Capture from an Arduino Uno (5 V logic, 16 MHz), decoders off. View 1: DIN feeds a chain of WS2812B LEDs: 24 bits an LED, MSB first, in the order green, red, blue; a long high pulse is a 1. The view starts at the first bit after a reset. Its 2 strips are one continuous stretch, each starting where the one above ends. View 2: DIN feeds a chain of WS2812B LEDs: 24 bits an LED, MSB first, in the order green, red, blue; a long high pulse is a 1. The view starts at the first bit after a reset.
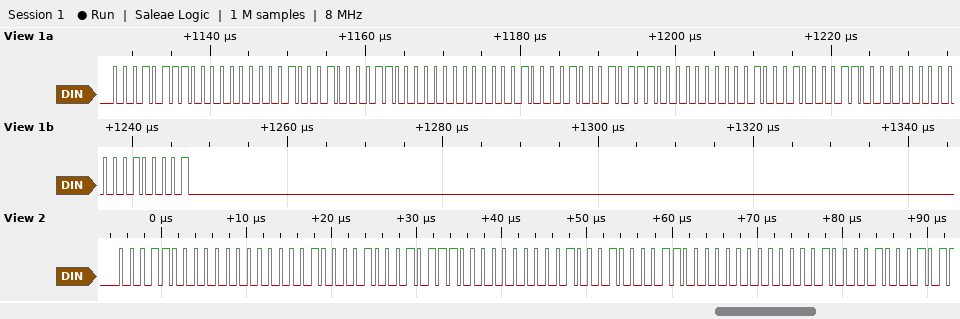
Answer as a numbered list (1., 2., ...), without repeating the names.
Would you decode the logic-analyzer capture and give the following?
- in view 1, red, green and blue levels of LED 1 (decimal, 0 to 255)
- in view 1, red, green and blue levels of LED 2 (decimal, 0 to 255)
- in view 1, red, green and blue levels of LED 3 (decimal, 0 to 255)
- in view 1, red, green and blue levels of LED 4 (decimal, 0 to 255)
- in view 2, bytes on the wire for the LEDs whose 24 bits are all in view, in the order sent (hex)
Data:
1. 0, 23, 34
2. 0, 24, 33
3. 0, 23, 34
4. 0, 24, 33
5. 18 00 21 17 00 22 18 00 21
